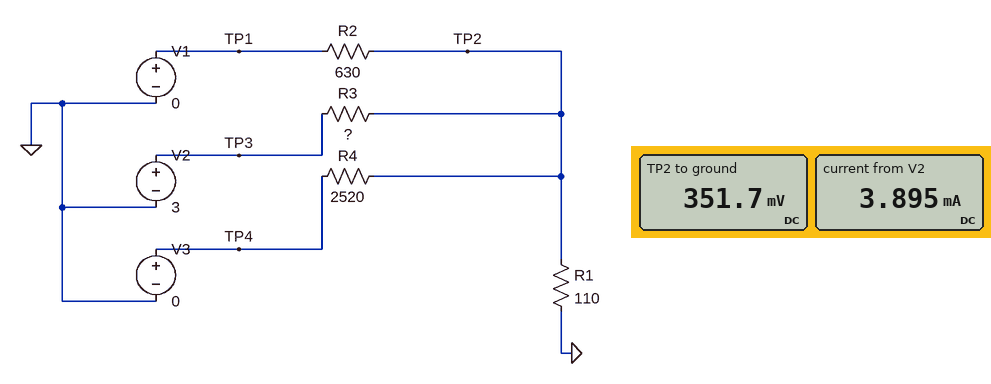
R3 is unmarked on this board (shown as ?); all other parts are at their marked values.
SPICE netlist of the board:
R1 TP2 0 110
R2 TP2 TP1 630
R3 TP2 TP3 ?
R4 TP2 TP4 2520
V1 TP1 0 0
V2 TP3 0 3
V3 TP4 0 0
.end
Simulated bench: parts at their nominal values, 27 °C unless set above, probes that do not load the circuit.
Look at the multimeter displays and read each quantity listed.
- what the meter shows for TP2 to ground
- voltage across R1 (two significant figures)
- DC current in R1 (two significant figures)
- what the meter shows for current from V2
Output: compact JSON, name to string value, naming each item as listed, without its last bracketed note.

{"what the meter shows for TP2 to ground": "351.7 mV", "voltage across R1": "350 mV", "DC current in R1": "3.2 mA", "what the meter shows for current from V2": "3.895 mA"}
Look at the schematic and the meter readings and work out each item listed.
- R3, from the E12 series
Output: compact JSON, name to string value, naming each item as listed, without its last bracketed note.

{"R3, from the E12 series": "680 Ω"}
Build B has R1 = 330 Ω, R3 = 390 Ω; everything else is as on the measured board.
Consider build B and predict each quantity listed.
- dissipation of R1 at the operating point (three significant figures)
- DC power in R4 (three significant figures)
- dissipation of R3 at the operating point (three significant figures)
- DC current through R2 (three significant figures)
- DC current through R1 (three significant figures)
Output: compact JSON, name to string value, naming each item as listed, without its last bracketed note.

{"dissipation of R1 at the operating point": "3.12 mW", "DC power in R4": "409 µW", "dissipation of R3 at the operating point": "10.1 mW", "DC current through R2": "1.61 mA", "DC current through R1": "3.08 mA"}
